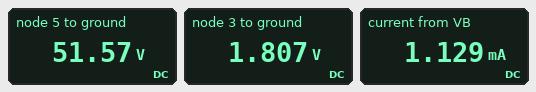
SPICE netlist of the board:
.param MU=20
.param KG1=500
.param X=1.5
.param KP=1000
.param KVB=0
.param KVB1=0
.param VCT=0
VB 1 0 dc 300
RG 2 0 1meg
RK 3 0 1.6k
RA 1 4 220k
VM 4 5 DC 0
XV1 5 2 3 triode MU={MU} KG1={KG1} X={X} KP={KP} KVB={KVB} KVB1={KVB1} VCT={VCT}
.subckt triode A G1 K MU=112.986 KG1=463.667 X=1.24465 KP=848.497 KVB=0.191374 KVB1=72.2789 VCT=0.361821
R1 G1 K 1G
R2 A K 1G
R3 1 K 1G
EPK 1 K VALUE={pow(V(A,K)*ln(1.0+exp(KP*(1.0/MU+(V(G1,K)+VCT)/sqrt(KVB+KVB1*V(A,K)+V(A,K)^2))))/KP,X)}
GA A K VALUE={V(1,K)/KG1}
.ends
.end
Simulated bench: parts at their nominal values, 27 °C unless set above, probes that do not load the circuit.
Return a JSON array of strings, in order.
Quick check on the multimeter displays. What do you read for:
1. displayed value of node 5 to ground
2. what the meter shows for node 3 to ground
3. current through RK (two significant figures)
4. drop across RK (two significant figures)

["51.57 V", "1.807 V", "1.1 mA", "1.8 V"]
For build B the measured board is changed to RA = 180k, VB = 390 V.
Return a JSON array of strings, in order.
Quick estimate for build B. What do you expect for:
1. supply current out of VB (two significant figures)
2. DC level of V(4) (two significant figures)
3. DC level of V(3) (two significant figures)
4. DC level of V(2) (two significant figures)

["1.7 mA", "77 V", "2.8 V", "2.8 mV"]
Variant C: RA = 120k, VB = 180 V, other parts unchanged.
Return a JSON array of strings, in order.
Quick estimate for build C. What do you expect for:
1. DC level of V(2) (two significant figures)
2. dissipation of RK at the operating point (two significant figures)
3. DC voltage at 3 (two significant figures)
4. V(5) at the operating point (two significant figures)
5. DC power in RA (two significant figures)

["1.7 mV", "1.9 mW", "1.7 V", "50 V", "140 mW"]
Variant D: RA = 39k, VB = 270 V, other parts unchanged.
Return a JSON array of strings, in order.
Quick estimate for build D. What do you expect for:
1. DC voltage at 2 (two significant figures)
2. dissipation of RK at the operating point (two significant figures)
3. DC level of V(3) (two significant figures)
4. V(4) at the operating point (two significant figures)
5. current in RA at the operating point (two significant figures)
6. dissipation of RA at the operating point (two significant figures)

["5.3 mV", "18 mW", "5.3 V", "140 V", "3.3 mA", "430 mW"]
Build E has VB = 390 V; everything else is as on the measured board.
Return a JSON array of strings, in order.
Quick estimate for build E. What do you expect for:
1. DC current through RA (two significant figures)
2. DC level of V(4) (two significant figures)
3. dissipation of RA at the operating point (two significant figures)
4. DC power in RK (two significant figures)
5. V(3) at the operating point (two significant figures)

["1.5 mA", "66 V", "480 mW", "3.5 mW", "2.4 V"]
